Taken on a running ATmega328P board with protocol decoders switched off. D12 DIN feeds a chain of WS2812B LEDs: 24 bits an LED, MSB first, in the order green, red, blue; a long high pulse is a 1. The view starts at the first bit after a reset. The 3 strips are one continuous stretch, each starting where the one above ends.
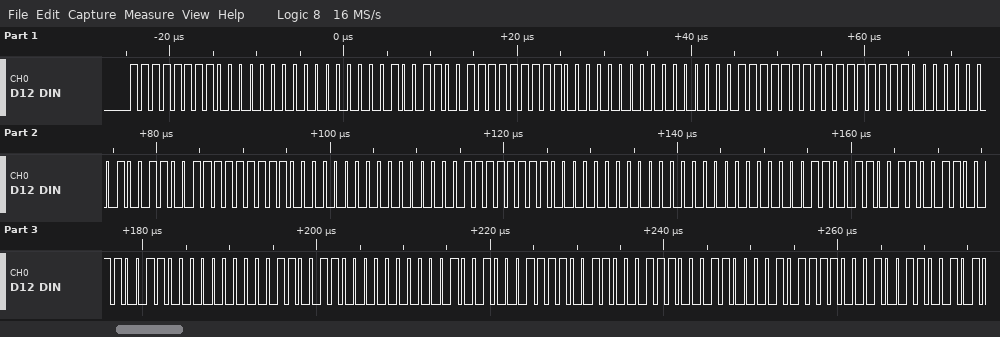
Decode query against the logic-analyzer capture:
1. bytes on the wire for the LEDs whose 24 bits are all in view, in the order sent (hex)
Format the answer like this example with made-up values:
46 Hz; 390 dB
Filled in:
FF 00 00 99 FF 00 00 FF FF 00 99 FF 00 00 FF 00 00 00 CC CC CC 00 CC 00 91 E6 38 C2 F1 32
